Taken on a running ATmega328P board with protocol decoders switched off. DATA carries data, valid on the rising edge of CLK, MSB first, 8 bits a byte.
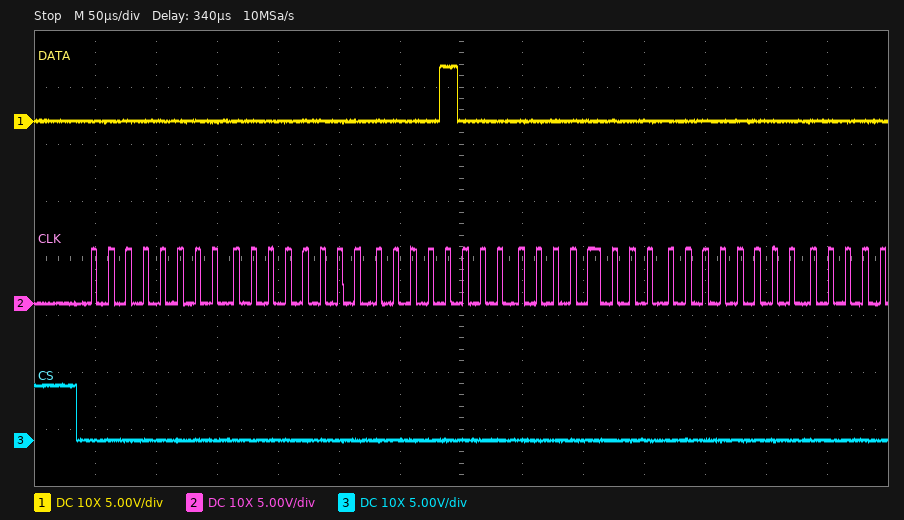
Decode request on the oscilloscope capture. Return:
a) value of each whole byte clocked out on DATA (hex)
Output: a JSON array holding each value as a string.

["00 00 08 00 00"]
